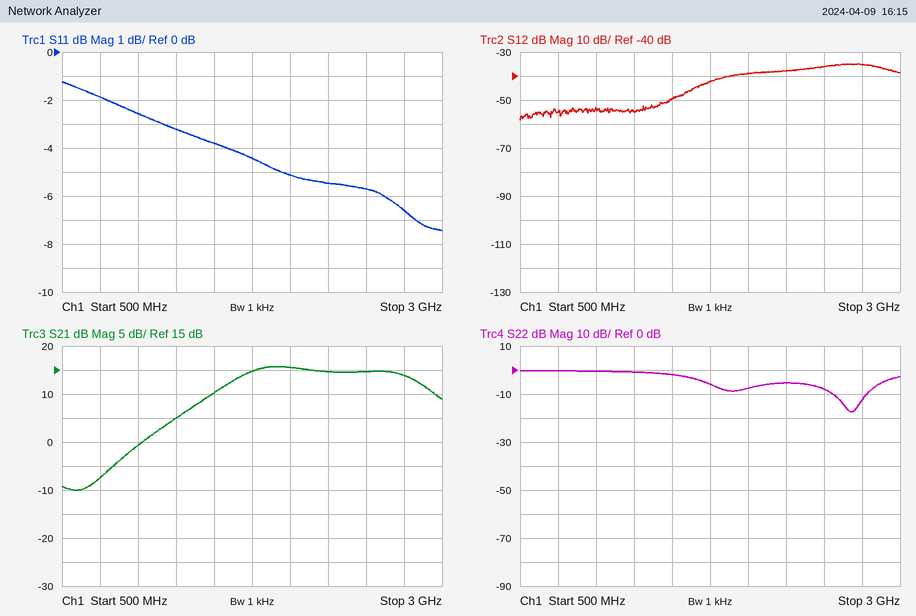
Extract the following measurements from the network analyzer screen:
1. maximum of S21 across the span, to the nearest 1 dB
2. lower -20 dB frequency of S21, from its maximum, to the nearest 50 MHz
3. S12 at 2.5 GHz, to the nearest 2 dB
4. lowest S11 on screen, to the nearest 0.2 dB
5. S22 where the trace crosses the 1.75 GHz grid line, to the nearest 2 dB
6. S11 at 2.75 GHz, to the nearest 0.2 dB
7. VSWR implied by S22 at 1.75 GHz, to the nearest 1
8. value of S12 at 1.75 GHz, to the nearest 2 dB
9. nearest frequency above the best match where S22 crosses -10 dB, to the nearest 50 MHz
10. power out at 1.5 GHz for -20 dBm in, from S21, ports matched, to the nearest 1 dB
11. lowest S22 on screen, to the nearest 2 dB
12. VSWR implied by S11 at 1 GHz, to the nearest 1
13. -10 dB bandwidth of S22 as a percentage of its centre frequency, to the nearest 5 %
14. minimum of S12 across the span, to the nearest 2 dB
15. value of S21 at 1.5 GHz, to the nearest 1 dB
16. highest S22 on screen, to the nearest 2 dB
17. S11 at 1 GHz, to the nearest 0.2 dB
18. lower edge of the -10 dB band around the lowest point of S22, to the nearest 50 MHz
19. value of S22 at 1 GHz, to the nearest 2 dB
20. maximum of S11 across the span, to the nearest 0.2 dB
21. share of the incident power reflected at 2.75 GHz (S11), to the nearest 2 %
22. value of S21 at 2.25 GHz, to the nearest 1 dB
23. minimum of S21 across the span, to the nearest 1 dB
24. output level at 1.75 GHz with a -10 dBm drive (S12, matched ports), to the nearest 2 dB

16 dB
850 MHz
-36 dB
-7.4 dB
-6 dB
-6.6 dB
3
-42 dB
2.80 GHz
-10 dBm
-18 dB
7
10 %
-58 dB
10 dB
0 dB
-2.6 dB
2.55 GHz
0 dB
-1.2 dB
22 %
15 dB
-10 dB
-52 dBm
